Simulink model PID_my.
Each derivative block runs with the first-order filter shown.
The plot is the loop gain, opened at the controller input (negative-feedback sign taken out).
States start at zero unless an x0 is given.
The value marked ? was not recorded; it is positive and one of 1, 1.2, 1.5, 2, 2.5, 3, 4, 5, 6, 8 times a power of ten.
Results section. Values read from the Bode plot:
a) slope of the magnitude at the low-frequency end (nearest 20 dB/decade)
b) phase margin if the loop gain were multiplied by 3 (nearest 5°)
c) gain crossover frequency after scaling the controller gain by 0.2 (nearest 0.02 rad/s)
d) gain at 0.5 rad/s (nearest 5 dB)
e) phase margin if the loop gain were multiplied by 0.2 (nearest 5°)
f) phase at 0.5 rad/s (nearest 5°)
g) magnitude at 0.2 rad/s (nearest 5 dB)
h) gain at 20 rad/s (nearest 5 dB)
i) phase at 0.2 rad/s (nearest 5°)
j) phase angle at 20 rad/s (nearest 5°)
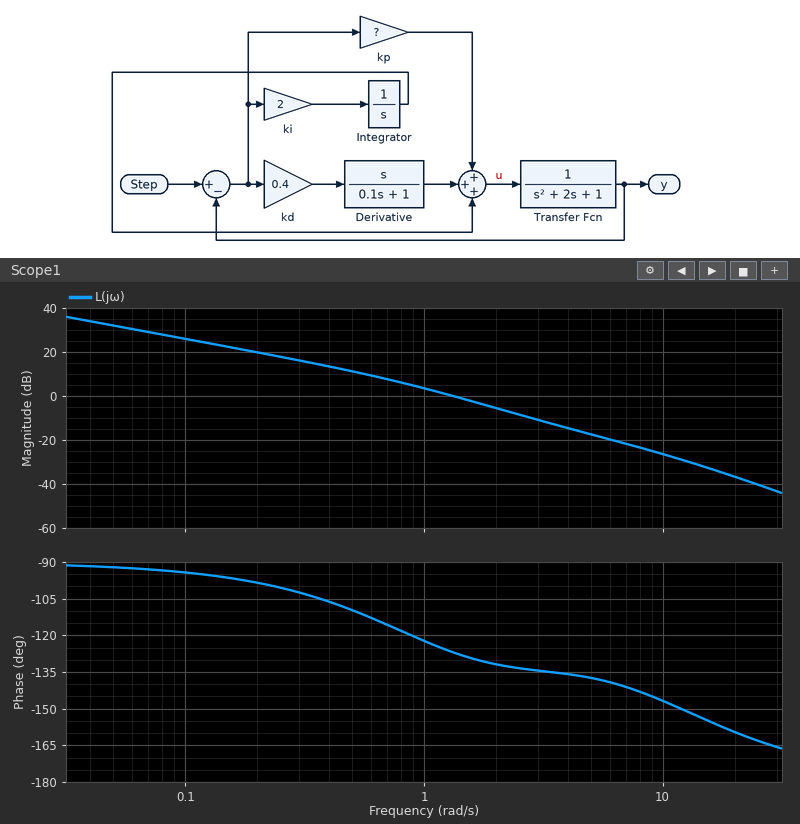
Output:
-20 dB/decade
45°
0.38 rad/s
10 dB
75°
-110°
20 dB
-35 dB
-100°
-160°
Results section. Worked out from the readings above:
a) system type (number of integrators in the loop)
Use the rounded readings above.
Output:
1
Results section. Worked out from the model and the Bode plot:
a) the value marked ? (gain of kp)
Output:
2.5
